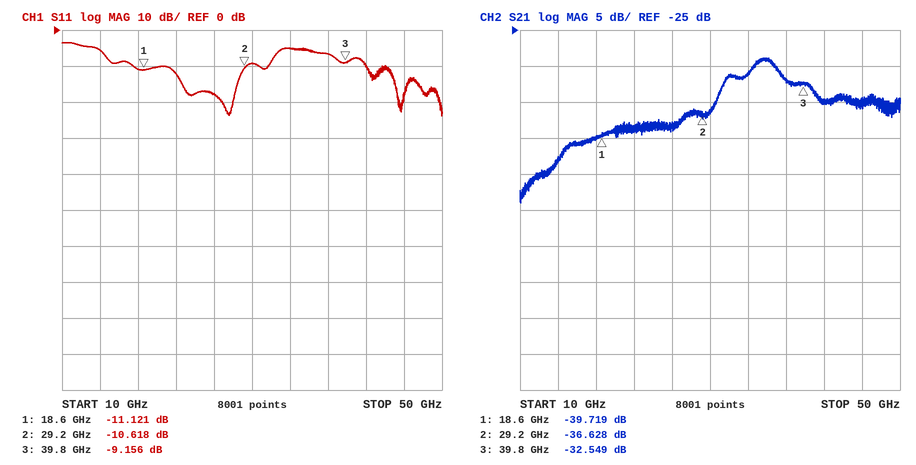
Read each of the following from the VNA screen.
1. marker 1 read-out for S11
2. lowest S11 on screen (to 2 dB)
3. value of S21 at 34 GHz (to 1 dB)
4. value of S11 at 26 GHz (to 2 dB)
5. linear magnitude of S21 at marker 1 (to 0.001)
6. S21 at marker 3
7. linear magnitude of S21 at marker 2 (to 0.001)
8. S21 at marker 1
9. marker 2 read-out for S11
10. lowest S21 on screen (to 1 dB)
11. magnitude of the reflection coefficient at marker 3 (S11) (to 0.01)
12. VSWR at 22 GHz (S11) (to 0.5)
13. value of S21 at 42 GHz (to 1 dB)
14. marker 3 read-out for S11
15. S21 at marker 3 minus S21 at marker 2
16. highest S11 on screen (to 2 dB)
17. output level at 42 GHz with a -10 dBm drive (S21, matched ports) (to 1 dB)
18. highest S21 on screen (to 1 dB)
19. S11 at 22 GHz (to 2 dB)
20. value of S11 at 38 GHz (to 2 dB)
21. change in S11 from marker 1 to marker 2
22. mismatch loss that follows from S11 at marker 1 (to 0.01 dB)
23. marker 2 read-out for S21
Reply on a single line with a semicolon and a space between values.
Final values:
-11.121 dB; -24 dB; -31 dB; -18 dB; 0.010; -32.549 dB; 0.015; -39.719 dB; -10.618 dB; -49 dB; 0.35; 1.5; -35 dB; -9.156 dB; 4.079 dB; -4 dB; -45 dBm; -29 dB; -12 dB; -6 dB; 0.503 dB; 0.35 dB; -36.628 dB
